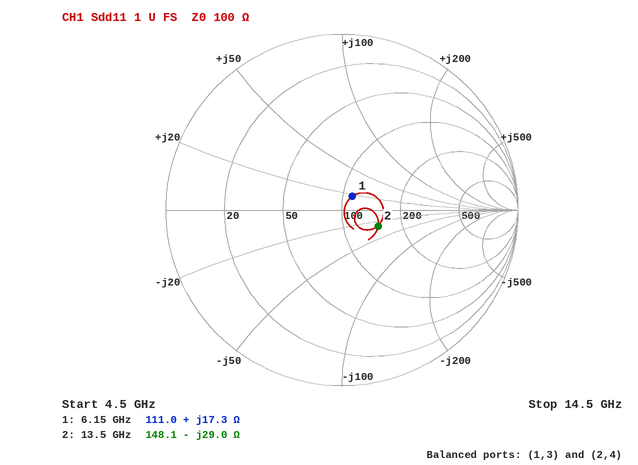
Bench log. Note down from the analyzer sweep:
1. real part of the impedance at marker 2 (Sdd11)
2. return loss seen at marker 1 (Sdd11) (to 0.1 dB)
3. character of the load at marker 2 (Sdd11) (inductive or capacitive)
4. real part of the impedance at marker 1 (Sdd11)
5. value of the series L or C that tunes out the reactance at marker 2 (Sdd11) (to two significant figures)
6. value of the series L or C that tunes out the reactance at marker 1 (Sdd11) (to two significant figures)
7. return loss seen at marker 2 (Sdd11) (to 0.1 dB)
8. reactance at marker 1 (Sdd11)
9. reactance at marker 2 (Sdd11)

148.1 Ω
20.3 dB
capacitive
111.0 Ω
340 pH
1.5 pF
13.0 dB
+17.3 Ω
-29.0 Ω
